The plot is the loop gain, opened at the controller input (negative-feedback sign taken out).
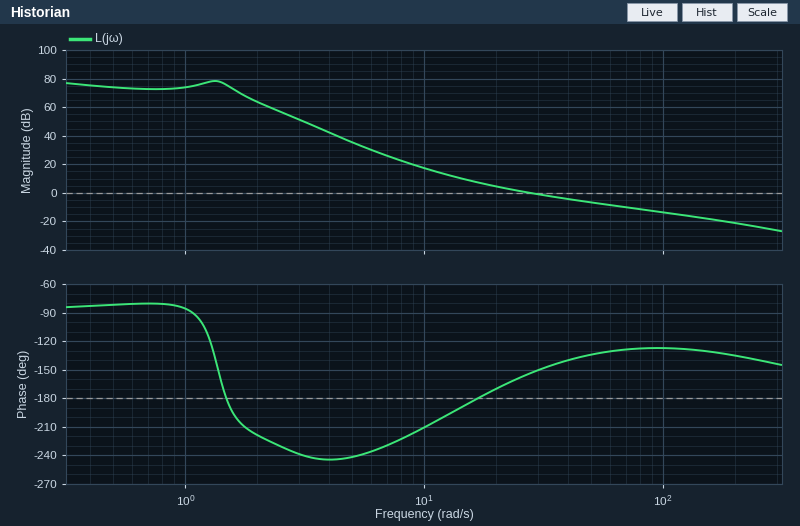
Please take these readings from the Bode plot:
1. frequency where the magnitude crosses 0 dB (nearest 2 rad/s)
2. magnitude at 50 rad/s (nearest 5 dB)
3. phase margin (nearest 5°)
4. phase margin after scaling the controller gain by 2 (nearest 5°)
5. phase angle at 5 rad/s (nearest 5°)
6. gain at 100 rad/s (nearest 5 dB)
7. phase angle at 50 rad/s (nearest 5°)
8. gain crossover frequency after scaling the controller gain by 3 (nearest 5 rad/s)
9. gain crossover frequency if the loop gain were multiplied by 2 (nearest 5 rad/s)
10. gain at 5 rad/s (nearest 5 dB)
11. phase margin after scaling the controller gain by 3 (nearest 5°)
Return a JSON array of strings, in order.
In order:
["28 rad/s", "-5 dB", "25°", "45°", "-240°", "-15 dB", "-135°", "65 rad/s", "45 rad/s", "35 dB", "50°"]
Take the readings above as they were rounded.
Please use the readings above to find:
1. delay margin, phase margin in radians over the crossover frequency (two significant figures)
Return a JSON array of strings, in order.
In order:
["0.016 s"]
